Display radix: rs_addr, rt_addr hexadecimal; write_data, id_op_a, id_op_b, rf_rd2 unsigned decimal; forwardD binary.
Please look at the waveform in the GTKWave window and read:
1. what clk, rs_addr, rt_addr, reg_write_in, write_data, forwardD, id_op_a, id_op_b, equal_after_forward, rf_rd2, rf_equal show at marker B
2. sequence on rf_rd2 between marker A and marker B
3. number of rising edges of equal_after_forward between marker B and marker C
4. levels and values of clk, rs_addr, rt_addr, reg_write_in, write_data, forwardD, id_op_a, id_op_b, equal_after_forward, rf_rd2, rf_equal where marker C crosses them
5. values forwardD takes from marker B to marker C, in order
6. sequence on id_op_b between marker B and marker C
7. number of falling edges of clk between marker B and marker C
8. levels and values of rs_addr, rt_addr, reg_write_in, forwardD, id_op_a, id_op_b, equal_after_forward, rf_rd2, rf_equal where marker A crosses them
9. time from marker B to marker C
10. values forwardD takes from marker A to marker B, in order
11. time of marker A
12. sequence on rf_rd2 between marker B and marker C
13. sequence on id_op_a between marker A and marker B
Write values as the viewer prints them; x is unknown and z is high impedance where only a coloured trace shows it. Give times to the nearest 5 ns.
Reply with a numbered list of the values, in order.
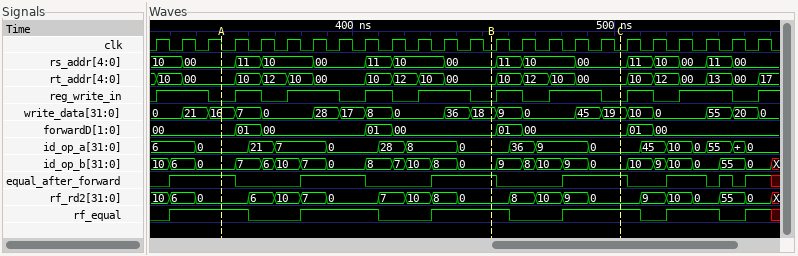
1. clk=0, rs_addr=00, rt_addr=00, reg_write_in=0, write_data=18, forwardD=00, id_op_a=0, id_op_b=0, equal_after_forward=1, rf_rd2=0, rf_equal=1
2. 0, 6, 10, 7, 0, 7, 10, 8, 0
3. 1
4. clk=0, rs_addr=00, rt_addr=00, reg_write_in=0, write_data=19, forwardD=00, id_op_a=0, id_op_b=0, equal_after_forward=1, rf_rd2=0, rf_equal=1
5. 00, 01, 00
6. 0, 9, 8, 10, 9, 0
7. 5
8. rs_addr=00, rt_addr=00, reg_write_in=0, forwardD=00, id_op_a=0, id_op_b=0, equal_after_forward=1, rf_rd2=0, rf_equal=1
9. 50 ns
10. 00, 01, 00, 01, 00
11. 350 ns
12. 0, 8, 10, 9, 0
13. 0, 21, 7, 0, 28, 8, 0
